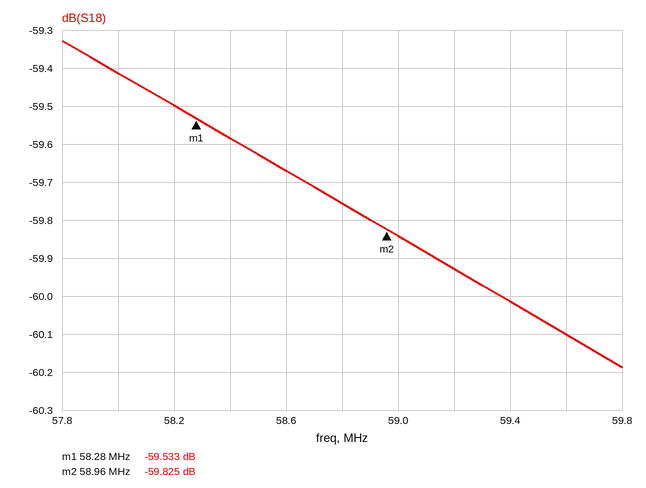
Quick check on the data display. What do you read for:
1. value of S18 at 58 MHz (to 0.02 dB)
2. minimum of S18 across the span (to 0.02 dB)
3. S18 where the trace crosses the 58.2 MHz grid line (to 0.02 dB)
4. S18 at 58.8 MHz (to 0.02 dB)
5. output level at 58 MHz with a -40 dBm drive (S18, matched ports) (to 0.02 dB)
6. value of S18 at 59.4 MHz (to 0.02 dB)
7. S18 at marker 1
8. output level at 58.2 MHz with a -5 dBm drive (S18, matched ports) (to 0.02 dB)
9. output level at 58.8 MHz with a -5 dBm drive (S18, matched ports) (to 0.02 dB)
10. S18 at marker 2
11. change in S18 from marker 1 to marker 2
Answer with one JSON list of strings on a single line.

["-59.42 dB", "-60.18 dB", "-59.50 dB", "-59.76 dB", "-99.42 dBm", "-60.02 dB", "-59.533 dB", "-64.50 dBm", "-64.76 dBm", "-59.825 dB", "-0.292 dB"]
